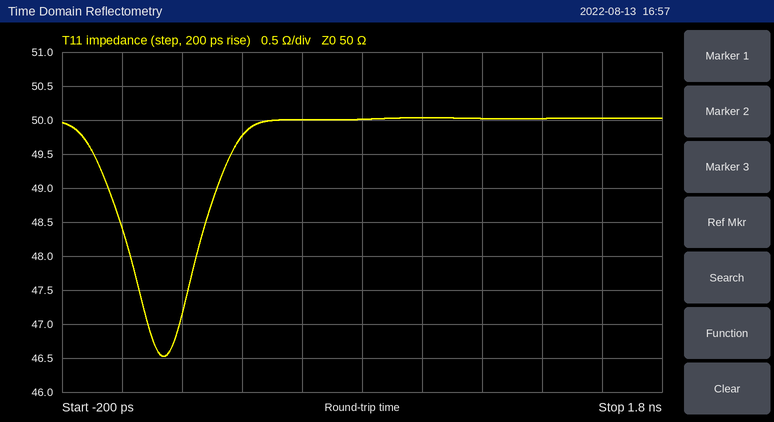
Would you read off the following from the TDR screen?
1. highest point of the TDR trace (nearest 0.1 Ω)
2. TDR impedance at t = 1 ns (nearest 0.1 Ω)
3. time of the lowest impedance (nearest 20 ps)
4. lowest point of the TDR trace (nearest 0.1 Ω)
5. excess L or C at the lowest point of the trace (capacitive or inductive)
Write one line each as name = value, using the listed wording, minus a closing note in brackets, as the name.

highest point of the TDR trace = 50.0 Ω
TDR impedance at t = 1 ns = 50.0 Ω
time of the lowest impedance = 140 ps
lowest point of the TDR trace = 46.5 Ω
excess L or C at the lowest point of the trace = capacitive
